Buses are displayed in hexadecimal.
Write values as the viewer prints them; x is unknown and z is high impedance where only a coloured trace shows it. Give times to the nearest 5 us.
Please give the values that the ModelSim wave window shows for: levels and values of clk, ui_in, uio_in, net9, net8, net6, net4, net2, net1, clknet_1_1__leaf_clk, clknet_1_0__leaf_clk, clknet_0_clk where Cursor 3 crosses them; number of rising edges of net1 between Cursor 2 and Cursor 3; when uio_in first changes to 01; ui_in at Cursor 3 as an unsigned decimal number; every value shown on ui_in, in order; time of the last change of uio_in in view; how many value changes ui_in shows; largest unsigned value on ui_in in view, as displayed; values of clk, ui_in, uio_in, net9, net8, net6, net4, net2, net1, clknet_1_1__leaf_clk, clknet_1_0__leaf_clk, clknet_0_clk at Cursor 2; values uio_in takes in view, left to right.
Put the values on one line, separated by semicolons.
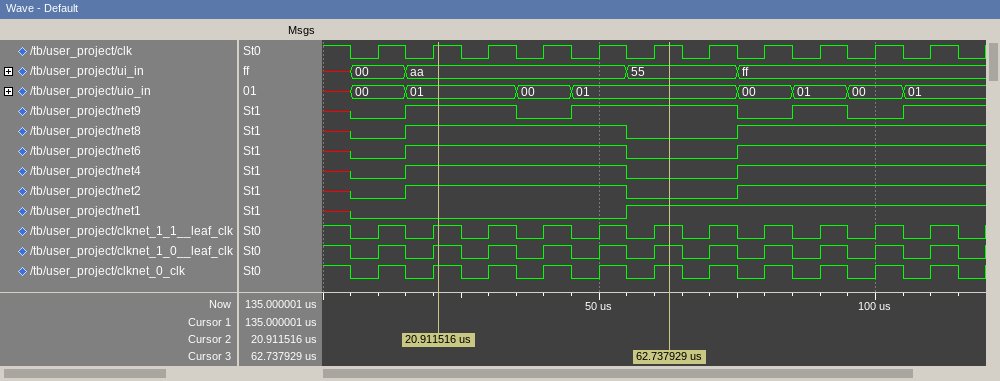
clk=1, ui_in=55, uio_in=01, net9=1, net8=0, net6=0, net4=0, net2=0, net1=1, clknet_1_1__leaf_clk=1, clknet_1_0__leaf_clk=1, clknet_0_clk=1; 1; 15 us; 85; x, 00, aa, 55, ff; 105 us; 4; ff; clk=1, ui_in=aa, uio_in=01, net9=1, net8=1, net6=1, net4=1, net2=1, net1=0, clknet_1_1__leaf_clk=1, clknet_1_0__leaf_clk=1, clknet_0_clk=1; x, 00, 01, 00, 01, 00, 01, 00, 01
